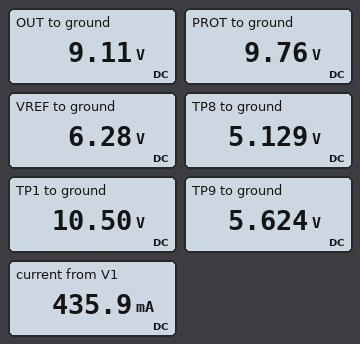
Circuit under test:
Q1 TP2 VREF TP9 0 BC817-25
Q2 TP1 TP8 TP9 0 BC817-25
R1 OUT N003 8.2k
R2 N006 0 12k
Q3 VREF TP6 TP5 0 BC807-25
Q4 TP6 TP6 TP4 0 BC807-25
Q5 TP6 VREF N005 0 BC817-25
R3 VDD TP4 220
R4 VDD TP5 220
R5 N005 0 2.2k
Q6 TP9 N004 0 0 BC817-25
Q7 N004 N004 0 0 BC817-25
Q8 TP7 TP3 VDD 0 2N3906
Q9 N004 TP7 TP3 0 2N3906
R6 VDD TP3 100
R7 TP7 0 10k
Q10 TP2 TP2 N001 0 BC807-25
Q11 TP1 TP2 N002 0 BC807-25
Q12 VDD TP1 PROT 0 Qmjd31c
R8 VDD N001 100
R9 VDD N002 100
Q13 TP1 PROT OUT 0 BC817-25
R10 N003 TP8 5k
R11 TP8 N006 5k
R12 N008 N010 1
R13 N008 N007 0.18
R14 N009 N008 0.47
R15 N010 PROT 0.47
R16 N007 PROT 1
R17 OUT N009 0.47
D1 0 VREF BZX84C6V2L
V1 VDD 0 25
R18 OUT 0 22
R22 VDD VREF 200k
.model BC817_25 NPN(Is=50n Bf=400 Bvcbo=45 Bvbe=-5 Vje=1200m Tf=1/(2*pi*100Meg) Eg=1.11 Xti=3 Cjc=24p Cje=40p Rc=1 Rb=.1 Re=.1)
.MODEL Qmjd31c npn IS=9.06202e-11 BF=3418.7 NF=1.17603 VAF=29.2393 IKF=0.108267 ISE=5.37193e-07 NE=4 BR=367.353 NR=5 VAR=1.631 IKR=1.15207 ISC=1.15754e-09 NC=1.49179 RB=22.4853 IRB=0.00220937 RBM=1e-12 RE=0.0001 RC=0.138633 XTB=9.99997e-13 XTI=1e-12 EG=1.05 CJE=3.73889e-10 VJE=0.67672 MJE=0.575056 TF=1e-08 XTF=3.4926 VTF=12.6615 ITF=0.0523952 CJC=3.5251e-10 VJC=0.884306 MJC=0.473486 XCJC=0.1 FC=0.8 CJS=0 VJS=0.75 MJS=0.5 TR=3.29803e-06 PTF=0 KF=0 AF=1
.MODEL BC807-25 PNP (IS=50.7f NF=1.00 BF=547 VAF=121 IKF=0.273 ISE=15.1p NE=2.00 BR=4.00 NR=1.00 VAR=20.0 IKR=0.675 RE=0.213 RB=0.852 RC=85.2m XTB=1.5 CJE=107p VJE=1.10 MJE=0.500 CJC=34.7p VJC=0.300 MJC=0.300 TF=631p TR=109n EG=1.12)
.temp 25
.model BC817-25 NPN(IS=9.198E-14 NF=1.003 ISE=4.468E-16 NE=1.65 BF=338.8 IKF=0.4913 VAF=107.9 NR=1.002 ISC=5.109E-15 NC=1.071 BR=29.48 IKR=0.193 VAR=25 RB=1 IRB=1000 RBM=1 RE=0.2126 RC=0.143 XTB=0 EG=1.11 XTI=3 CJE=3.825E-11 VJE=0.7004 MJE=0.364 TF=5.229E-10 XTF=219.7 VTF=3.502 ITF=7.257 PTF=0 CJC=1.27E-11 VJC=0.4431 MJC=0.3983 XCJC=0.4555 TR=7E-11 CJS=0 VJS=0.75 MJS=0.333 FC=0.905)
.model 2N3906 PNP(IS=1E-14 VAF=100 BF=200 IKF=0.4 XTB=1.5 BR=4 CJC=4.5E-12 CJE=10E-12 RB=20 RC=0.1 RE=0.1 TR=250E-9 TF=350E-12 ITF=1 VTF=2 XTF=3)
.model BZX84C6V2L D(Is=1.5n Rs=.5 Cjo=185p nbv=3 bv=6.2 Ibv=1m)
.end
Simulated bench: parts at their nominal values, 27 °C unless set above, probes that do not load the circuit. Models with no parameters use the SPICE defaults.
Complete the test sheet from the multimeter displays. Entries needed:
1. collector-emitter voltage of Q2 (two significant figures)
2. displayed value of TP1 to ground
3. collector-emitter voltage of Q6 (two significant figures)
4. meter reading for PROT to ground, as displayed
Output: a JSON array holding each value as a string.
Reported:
["4.9 V", "10.50 V", "5.6 V", "9.76 V"]
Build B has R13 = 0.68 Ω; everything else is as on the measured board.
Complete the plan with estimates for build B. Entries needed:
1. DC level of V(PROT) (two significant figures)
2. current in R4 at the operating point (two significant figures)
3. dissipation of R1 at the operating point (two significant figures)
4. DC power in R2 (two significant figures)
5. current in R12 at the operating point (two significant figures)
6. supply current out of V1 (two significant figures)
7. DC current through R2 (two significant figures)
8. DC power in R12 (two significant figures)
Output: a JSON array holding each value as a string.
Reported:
["9.1 V", "2.6 mA", "640 µW", "940 µW", "200 mA", "410 mA", "280 µA", "41 mW"]
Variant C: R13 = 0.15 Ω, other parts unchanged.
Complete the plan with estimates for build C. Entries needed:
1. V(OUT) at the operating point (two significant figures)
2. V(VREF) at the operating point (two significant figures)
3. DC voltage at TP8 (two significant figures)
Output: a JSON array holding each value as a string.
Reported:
["9.2 V", "6.3 V", "5.2 V"]
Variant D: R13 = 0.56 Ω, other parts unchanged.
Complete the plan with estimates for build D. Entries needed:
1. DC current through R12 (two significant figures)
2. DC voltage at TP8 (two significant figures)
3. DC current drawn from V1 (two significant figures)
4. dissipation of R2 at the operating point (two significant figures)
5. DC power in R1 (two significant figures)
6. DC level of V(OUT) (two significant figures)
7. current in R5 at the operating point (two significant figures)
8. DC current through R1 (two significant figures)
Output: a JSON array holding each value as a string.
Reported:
["200 mA", "4.8 V", "410 mA", "970 µW", "660 µW", "8.6 V", "2.6 mA", "280 µA"]
